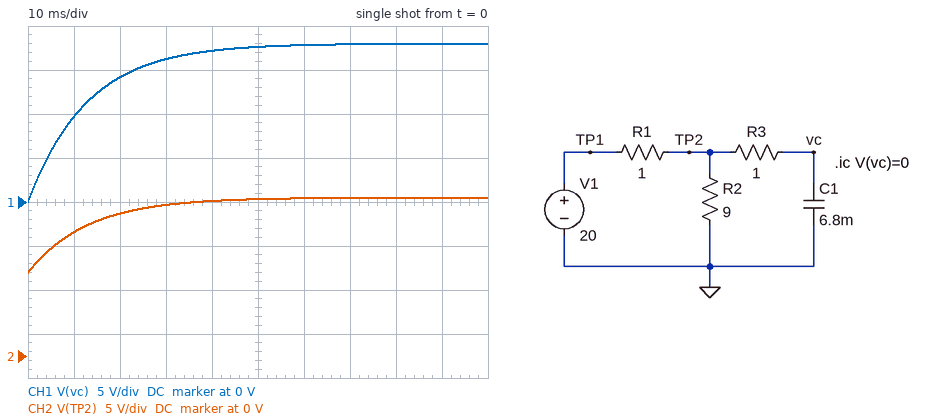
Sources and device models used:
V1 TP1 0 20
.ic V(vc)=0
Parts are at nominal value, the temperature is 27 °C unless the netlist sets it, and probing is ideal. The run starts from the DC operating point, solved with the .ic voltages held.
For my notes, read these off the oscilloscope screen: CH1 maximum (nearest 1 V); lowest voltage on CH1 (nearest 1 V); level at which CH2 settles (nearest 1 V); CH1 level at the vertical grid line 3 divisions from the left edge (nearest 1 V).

18 V
0 V
18 V
16 V
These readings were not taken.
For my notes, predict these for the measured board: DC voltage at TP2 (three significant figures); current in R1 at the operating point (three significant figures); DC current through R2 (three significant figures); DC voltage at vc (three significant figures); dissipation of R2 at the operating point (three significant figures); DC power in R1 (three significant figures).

18.0 V
2.00 A
2.00 A
18.0 V
36.0 W
4.00 W
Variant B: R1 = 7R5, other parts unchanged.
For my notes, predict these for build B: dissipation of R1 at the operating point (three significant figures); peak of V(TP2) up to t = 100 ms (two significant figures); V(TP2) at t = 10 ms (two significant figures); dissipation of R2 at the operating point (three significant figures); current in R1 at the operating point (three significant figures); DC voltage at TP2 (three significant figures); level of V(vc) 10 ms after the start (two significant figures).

11.0 W
10 V
4.3 V
13.2 W
1.21 A
10.9 V
2.7 V
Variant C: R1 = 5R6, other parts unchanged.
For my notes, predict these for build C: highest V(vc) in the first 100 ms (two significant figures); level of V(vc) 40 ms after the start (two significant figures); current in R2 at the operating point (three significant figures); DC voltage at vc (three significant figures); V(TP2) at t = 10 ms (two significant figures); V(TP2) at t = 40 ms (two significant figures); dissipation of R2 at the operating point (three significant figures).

12 V
9.0 V
1.37 A
12.3 V
5.5 V
9.8 V
16.9 W
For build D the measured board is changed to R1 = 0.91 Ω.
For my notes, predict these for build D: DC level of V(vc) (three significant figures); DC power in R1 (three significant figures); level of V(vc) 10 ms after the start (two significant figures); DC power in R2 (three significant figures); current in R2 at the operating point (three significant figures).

18.2 V
3.71 W
10 V
36.7 W
2.02 A
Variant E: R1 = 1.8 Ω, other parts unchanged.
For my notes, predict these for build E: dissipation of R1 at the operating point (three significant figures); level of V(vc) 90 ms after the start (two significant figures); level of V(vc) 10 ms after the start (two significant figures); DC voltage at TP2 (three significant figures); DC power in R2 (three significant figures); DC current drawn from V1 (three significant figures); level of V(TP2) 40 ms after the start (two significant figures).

6.17 W
17 V
7.4 V
16.7 V
30.9 W
1.85 A
16 V
